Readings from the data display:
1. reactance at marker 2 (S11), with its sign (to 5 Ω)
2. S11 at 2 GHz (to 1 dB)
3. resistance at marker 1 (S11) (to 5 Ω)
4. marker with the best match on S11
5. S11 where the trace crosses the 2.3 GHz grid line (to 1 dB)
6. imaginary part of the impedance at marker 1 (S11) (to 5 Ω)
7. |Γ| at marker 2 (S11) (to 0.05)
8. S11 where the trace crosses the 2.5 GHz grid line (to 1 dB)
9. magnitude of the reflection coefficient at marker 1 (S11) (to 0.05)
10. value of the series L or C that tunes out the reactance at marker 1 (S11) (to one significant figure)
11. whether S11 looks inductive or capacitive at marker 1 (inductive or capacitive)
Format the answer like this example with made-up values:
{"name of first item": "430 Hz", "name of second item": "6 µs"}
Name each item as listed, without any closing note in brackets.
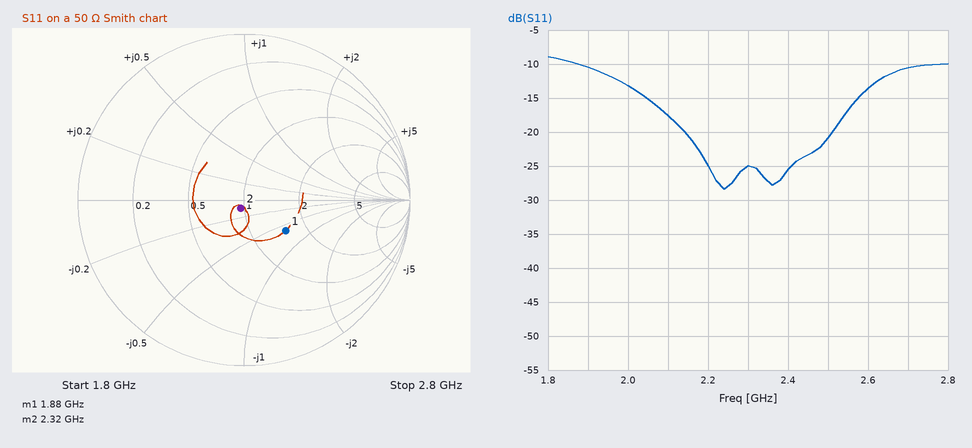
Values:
{"reactance at marker 2 (S11), with its sign": "-5 Ω", "S11 at 2 GHz": "-13 dB", "resistance at marker 1 (S11)": "75 Ω", "marker with the best match on S11": "marker 2", "S11 where the trace crosses the 2.3 GHz grid line": "-25 dB", "imaginary part of the impedance at marker 1 (S11)": "-30 Ω", "|Γ| at marker 2 (S11)": "0.05", "S11 where the trace crosses the 2.5 GHz grid line": "-21 dB", "magnitude of the reflection coefficient at marker 1 (S11)": "0.30", "value of the series L or C that tunes out the reactance at marker 1 (S11)": "3 nH", "whether S11 looks inductive or capacitive at marker 1": "capacitive"}
